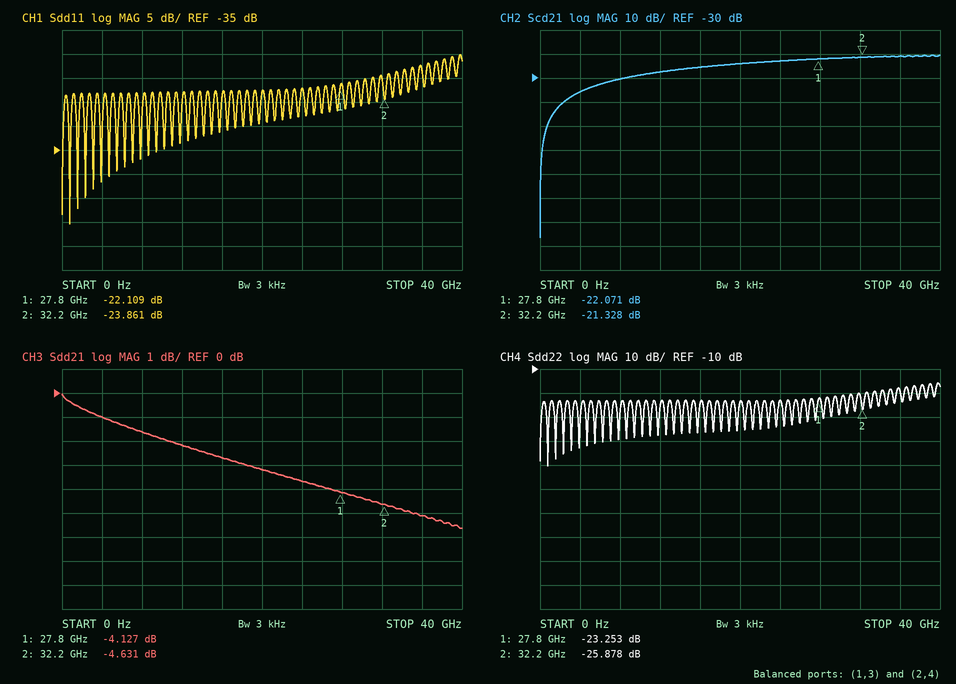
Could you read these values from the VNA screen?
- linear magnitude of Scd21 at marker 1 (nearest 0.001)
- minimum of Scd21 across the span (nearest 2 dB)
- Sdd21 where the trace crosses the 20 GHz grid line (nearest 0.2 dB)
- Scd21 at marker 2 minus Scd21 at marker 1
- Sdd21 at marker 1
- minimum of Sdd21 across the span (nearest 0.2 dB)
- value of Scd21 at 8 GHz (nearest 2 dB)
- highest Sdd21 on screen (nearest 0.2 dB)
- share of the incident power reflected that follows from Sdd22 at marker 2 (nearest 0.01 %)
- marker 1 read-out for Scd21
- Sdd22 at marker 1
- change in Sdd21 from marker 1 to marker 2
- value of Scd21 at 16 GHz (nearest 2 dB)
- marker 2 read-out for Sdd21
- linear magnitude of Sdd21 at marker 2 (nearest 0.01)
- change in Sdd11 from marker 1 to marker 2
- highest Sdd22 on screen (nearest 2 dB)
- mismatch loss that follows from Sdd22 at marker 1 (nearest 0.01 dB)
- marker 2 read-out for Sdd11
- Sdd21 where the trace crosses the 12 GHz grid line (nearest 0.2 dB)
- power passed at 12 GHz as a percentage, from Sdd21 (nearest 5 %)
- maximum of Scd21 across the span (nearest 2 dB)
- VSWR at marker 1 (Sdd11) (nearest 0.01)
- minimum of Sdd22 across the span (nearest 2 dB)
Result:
0.079
-96 dB
-3.2 dB
0.743 dB
-4.127 dB
-5.6 dB
-30 dB
0.0 dB
0.26 %
-22.071 dB
-23.253 dB
-0.504 dB
-26 dB
-4.631 dB
0.59
-1.752 dB
-16 dB
0.02 dB
-23.861 dB
-2.2 dB
60 %
-20 dB
1.17
-50 dB
